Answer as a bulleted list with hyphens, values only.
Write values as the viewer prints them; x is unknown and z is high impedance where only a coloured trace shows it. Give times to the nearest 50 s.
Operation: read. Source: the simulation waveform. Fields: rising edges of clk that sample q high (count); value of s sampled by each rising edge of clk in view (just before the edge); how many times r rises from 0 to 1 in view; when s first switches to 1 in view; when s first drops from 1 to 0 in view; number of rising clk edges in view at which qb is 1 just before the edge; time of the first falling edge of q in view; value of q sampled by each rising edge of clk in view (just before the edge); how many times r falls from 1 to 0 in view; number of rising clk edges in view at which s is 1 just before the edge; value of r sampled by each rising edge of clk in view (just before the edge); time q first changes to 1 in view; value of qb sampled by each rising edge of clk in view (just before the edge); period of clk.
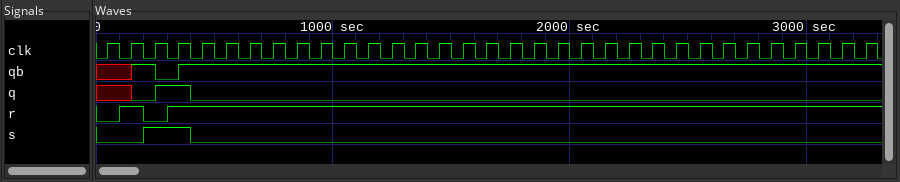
- 1
- 0 0 1 1 0 0 0 0 0 0 0 0 0 0 0 0 0 0 0 0 0 0 0 0 0 0 0 0 0 0 0 0 0
- 2
- 200 s
- 400 s
- 30
- 400 s
- x x 0 1 0 0 0 0 0 0 0 0 0 0 0 0 0 0 0 0 0 0 0 0 0 0 0 0 0 0 0 0 0
- 1
- 2
- 0 1 0 1 1 1 1 1 1 1 1 1 1 1 1 1 1 1 1 1 1 1 1 1 1 1 1 1 1 1 1 1 1
- 250 s
- x x 1 0 1 1 1 1 1 1 1 1 1 1 1 1 1 1 1 1 1 1 1 1 1 1 1 1 1 1 1 1 1
- 100 s
